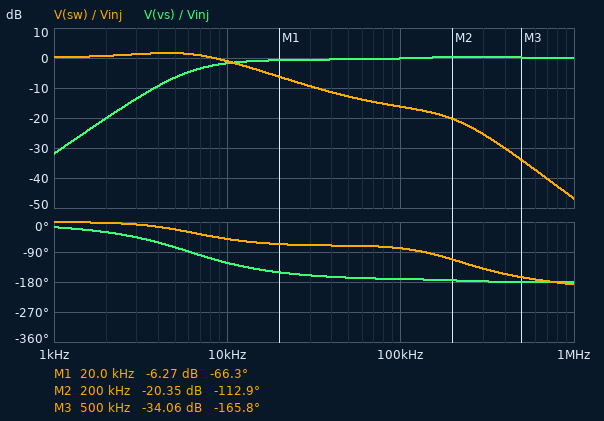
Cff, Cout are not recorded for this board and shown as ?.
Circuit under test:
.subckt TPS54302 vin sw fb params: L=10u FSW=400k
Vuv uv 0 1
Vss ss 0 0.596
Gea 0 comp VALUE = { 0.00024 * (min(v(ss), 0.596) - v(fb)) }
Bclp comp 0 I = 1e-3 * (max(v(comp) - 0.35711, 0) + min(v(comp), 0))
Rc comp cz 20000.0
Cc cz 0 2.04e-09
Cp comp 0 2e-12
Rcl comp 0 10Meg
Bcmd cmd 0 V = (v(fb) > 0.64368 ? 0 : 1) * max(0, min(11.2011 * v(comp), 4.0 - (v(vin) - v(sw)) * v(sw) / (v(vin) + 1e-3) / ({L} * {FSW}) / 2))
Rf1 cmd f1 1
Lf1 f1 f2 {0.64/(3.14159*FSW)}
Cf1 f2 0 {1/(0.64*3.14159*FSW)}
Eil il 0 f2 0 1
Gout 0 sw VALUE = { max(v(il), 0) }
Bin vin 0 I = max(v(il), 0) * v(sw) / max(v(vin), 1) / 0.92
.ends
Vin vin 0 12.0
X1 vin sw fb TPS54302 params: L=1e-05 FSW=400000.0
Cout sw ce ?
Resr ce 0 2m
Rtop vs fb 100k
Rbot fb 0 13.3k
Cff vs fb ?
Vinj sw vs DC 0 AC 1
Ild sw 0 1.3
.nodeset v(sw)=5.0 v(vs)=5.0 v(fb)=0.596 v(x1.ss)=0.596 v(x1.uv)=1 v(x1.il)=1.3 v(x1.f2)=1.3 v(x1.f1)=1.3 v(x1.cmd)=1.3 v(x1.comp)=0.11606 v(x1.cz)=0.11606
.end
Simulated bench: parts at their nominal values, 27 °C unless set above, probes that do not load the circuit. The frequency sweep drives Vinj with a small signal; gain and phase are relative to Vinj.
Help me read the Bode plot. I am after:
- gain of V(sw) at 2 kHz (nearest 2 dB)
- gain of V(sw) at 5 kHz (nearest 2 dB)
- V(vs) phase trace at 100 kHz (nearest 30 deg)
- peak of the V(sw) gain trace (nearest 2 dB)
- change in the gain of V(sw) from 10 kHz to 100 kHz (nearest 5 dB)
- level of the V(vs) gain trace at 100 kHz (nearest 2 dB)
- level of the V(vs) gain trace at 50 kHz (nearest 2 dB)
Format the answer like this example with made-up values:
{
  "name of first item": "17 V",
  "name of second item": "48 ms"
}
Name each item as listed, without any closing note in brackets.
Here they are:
{
  "gain of V(sw) at 2 kHz": "0 dB",
  "gain of V(sw) at 5 kHz": "2 dB",
  "V(vs) phase trace at 100 kHz": "-180 deg",
  "peak of the V(sw) gain trace": "2 dB",
  "change in the gain of V(sw) from 10 kHz to 100 kHz": "-15 dB",
  "level of the V(vs) gain trace at 100 kHz": "0 dB",
  "level of the V(vs) gain trace at 50 kHz": "0 dB"
}
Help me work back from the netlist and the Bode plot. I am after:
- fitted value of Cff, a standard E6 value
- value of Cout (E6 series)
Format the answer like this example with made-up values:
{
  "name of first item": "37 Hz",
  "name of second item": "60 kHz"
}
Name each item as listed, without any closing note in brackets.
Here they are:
{
  "fitted value of Cff, a standard E6 value": "22 pF",
  "value of Cout": "100 µF"
}
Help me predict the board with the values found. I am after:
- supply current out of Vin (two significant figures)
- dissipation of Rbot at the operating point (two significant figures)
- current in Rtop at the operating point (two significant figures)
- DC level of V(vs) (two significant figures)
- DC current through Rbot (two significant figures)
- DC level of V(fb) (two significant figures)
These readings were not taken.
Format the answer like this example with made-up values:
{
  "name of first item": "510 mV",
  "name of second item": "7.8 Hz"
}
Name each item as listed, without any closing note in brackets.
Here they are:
{
  "supply current out of Vin": "600 mA",
  "dissipation of Rbot at the operating point": "27 µW",
  "current in Rtop at the operating point": "45 µA",
  "DC level of V(vs)": "5.1 V",
  "DC current through Rbot": "45 µA",
  "DC level of V(fb)": "600 mV"
}
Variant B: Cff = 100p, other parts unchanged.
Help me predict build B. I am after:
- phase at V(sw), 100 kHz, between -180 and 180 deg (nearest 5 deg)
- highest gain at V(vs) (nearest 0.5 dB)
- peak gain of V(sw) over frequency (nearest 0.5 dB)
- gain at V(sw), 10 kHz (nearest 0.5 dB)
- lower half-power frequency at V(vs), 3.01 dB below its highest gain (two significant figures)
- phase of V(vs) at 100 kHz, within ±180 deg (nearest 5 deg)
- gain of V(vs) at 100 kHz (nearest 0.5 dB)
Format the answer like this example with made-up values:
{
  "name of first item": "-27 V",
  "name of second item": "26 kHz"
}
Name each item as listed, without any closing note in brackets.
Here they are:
{
  "phase at V(sw), 100 kHz, between -180 and 180 deg": "-65 deg",
  "highest gain at V(vs)": "1.5 dB",
  "peak gain of V(sw) over frequency": "1.0 dB",
  "gain at V(sw), 10 kHz": "-2.5 dB",
  "lower half-power frequency at V(vs), 3.01 dB below its highest gain": "90 kHz",
  "phase of V(vs) at 100 kHz, within ±180 deg": "-155 deg",
  "gain of V(vs) at 100 kHz": "-1.0 dB"
}
